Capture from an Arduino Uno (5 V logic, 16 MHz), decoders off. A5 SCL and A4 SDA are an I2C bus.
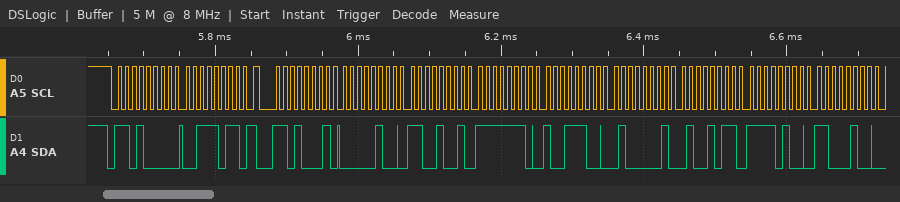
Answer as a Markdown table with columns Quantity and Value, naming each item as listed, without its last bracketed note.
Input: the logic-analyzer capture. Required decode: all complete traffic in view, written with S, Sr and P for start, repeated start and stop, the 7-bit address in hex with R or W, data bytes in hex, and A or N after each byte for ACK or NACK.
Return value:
| Quantity | Value |
|---|---|
| all complete traffic in view, written with S, Sr and P for start, repeated start and stop, the 7-bit address in hex with R or W, data bytes in hex, and A or N after each byte for ACK or NACK | S 68W A 3B A Sr 68R A 04 A C9 A FE A 9C A 41 A 4B A F4 A C4 A |
